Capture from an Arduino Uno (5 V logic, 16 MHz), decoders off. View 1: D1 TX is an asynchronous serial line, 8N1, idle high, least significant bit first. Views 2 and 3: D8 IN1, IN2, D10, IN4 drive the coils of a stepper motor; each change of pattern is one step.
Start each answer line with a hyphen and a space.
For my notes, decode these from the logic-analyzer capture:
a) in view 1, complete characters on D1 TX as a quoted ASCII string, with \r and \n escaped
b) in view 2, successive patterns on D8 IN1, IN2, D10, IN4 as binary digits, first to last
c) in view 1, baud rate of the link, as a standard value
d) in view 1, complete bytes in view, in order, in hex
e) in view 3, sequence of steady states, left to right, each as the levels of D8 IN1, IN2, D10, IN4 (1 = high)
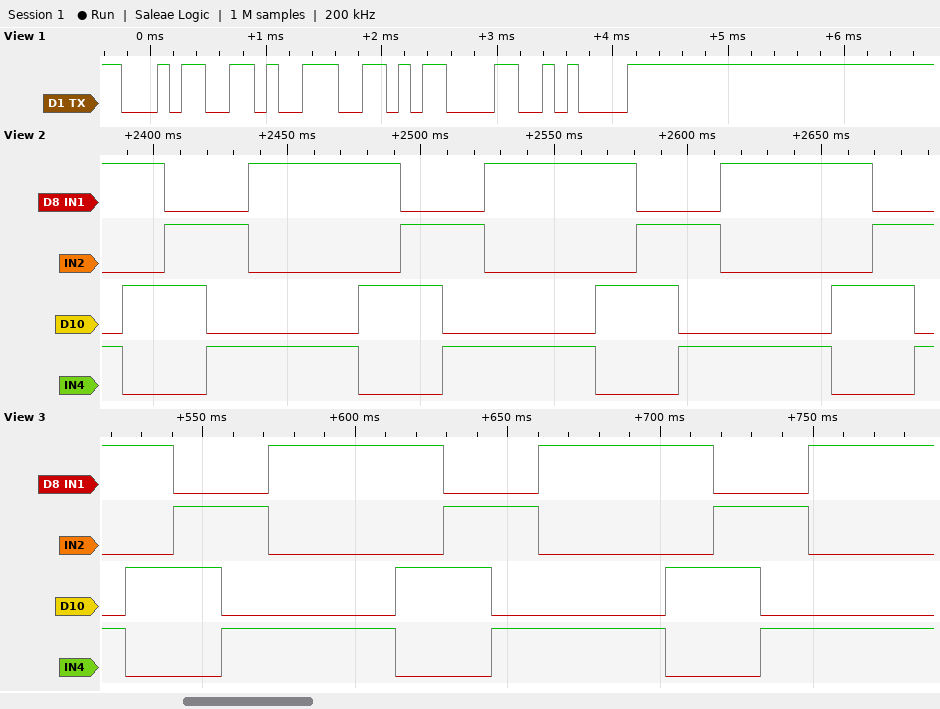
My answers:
- "49\r\n"
- 1001 1010 0110 0101 1001 1010 0110 0101 1001 1010 0110 0101 1001 1010 0110 0101
- 9600 baud
- 34 39 0D 0A
- 1001 1010 0110 0101 1001 1010 0110 0101 1001 1010 0110 0101 1001
